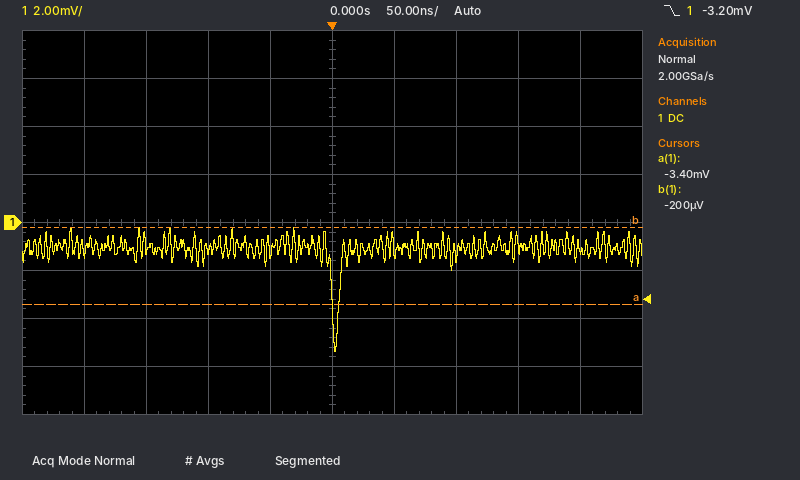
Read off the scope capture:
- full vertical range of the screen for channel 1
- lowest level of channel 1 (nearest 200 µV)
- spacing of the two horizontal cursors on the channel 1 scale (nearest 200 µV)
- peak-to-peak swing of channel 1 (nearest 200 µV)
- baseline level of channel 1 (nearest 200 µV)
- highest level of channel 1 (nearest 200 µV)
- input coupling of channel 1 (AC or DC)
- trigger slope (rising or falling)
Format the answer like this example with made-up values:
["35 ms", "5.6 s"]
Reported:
["16 mV", "-5.4 mV", "3.2 mV", "5.2 mV", "-1.0 mV", "-200 µV", "DC", "falling"]
